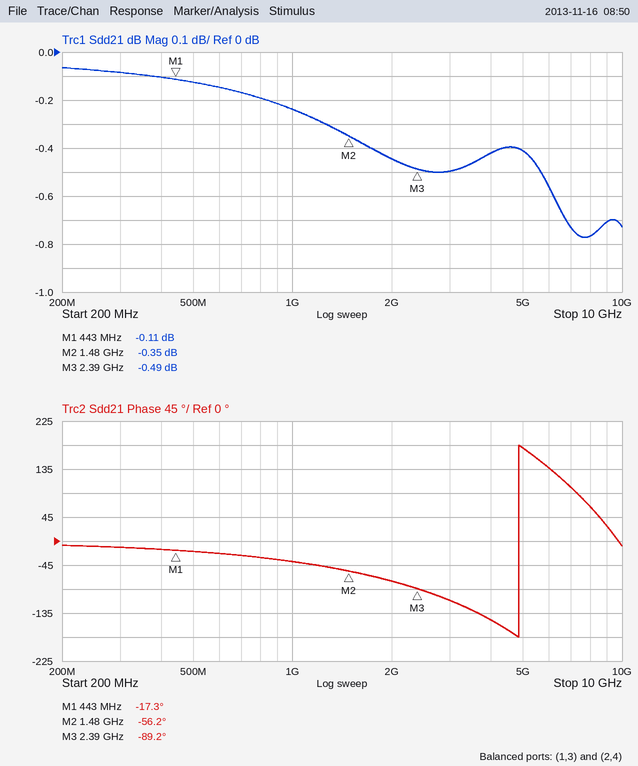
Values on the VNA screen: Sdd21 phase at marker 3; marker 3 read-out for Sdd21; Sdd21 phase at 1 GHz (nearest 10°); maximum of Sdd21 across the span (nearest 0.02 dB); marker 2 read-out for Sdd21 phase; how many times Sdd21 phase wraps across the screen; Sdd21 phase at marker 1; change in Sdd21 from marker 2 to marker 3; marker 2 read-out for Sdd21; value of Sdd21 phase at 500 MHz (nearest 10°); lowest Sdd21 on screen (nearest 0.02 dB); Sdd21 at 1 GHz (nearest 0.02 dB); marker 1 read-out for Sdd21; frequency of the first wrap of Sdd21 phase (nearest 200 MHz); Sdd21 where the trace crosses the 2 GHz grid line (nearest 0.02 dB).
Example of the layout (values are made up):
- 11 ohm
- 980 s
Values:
- -89.2°
- -0.49 dB
- -40°
- -0.06 dB
- -56.2°
- 1
- -17.3°
- -0.14 dB
- -0.35 dB
- -20°
- -0.78 dB
- -0.24 dB
- -0.11 dB
- 4.8 GHz
- -0.44 dB
